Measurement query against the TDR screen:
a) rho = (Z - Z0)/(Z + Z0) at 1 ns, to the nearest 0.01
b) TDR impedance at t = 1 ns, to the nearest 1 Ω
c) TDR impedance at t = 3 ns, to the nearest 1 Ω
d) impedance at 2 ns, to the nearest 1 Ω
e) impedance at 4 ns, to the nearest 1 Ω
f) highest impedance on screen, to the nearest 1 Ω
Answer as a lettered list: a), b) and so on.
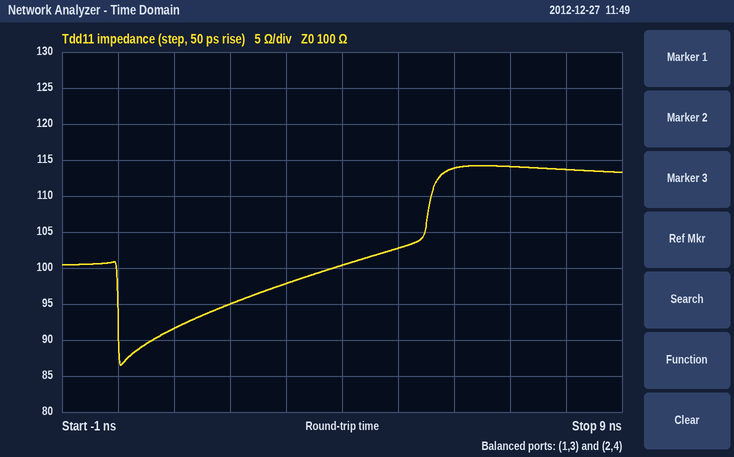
a) -0.04
b) 92 Ω
c) 98 Ω
d) 95 Ω
e) 100 Ω
f) 114 Ω
